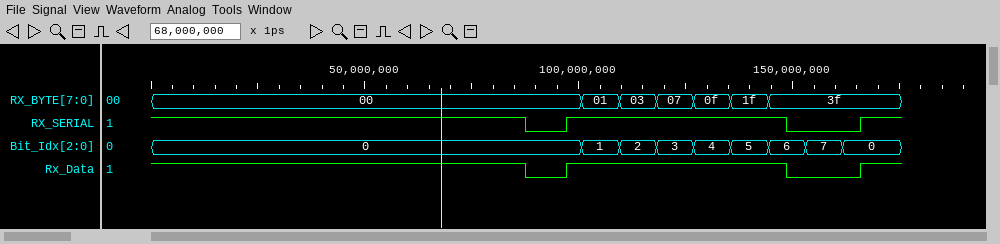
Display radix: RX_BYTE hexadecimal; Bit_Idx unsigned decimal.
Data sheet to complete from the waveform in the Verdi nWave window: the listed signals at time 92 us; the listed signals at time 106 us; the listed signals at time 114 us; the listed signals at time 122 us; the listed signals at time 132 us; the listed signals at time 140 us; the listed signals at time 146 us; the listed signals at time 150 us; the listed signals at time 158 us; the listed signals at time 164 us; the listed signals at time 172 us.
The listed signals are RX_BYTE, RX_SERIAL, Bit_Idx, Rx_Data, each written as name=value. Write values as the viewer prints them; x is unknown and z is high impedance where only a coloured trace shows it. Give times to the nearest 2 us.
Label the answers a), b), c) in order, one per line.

a) RX_BYTE=00, RX_SERIAL=0, Bit_Idx=0, Rx_Data=0
b) RX_BYTE=01, RX_SERIAL=1, Bit_Idx=1, Rx_Data=1
c) RX_BYTE=03, RX_SERIAL=1, Bit_Idx=2, Rx_Data=1
d) RX_BYTE=07, RX_SERIAL=1, Bit_Idx=3, Rx_Data=1
e) RX_BYTE=0f, RX_SERIAL=1, Bit_Idx=4, Rx_Data=1
f) RX_BYTE=1f, RX_SERIAL=1, Bit_Idx=5, Rx_Data=1
g) RX_BYTE=3f, RX_SERIAL=1, Bit_Idx=6, Rx_Data=1
h) RX_BYTE=3f, RX_SERIAL=0, Bit_Idx=6, Rx_Data=0
i) RX_BYTE=3f, RX_SERIAL=0, Bit_Idx=7, Rx_Data=0
j) RX_BYTE=3f, RX_SERIAL=0, Bit_Idx=0, Rx_Data=0
k) RX_BYTE=3f, RX_SERIAL=1, Bit_Idx=0, Rx_Data=1
